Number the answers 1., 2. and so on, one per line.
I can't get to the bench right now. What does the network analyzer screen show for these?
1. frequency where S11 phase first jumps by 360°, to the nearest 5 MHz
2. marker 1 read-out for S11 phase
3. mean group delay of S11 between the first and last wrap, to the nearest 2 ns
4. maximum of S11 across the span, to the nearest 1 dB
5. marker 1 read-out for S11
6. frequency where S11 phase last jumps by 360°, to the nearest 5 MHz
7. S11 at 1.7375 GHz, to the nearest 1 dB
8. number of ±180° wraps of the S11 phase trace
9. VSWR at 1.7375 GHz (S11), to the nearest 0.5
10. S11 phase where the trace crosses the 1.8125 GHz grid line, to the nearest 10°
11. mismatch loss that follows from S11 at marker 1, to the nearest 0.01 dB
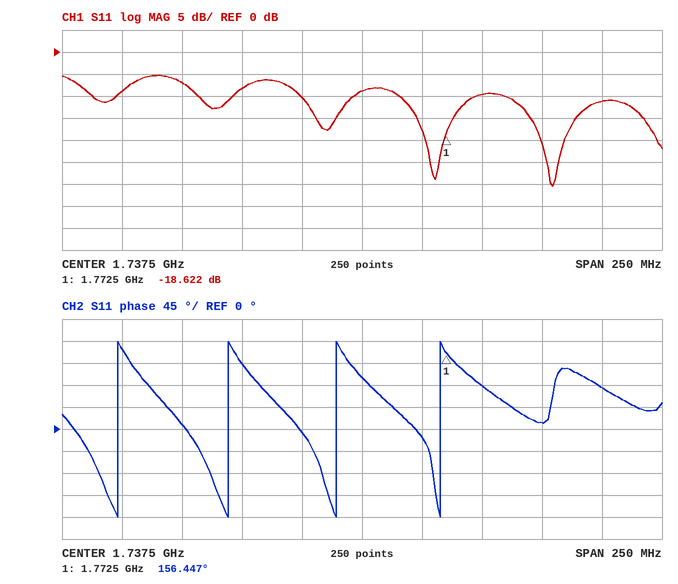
1. 1.635 GHz
2. 156.447°
3. 22 ns
4. -5 dB
5. -18.622 dB
6. 1.770 GHz
7. -9 dB
8. 4
9. 2.0
10. 10°
11. 0.06 dB
